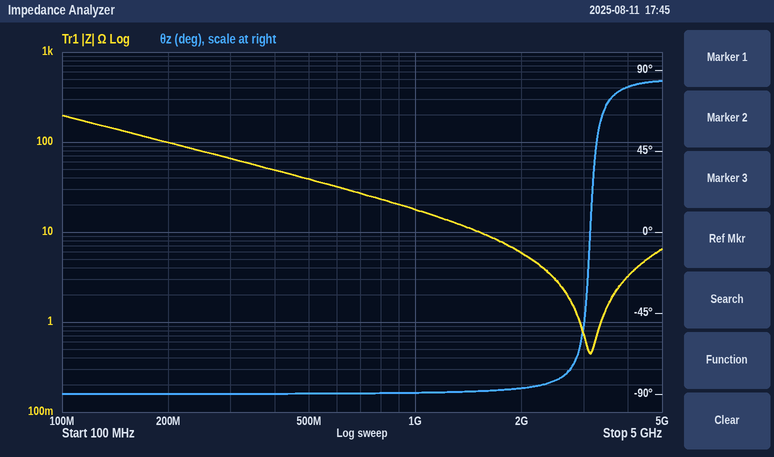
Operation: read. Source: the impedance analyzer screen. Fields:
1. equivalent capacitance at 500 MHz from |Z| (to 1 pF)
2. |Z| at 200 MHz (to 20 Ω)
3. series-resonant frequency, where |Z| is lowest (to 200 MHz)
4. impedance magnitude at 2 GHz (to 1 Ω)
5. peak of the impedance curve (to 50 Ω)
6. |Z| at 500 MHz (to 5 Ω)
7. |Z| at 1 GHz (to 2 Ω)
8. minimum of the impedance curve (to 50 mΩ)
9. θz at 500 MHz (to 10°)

8 pF
100 Ω
3.2 GHz
6 Ω
200 Ω
40 Ω
18 Ω
450 mΩ
-90°
